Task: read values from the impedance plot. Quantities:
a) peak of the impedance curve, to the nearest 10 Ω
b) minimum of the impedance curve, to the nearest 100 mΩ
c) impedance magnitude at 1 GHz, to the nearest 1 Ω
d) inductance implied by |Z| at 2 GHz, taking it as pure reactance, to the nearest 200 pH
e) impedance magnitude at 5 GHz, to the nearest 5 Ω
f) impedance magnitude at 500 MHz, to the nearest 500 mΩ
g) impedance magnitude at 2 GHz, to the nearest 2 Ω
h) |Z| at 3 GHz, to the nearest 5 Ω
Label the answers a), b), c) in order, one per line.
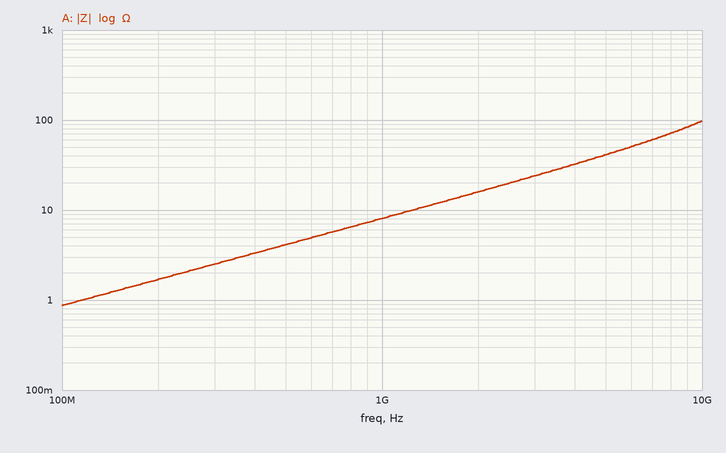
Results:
a) 100 Ω
b) 900 mΩ
c) 8 Ω
d) 1.2 nH
e) 40 Ω
f) 4.0 Ω
g) 16 Ω
h) 25 Ω
